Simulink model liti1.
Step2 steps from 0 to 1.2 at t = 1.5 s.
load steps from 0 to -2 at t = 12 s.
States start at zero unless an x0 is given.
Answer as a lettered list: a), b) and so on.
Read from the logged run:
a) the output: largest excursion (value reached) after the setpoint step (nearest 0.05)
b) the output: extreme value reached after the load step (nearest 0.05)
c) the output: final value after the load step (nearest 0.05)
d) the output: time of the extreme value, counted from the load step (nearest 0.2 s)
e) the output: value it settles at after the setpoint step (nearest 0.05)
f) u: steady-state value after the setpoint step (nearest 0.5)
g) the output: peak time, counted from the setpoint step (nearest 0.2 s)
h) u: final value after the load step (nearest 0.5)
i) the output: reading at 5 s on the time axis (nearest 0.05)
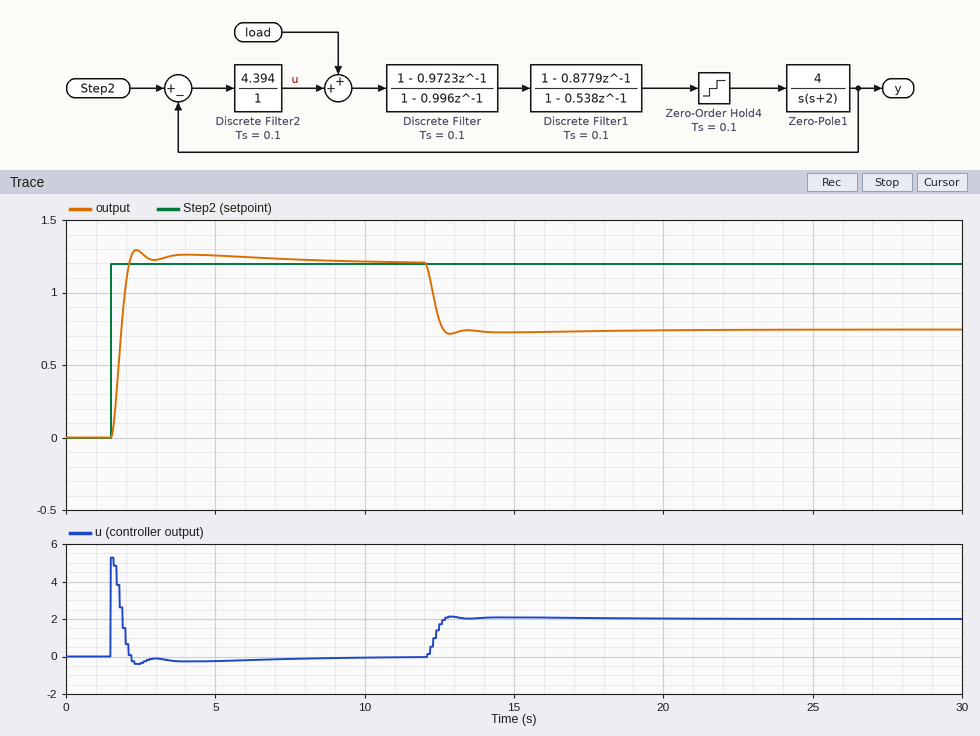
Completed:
a) 1.30
b) 0.70
c) 0.75
d) 0.8 s
e) 1.20
f) 0.0
g) 0.8 s
h) 2.0
i) 1.25
